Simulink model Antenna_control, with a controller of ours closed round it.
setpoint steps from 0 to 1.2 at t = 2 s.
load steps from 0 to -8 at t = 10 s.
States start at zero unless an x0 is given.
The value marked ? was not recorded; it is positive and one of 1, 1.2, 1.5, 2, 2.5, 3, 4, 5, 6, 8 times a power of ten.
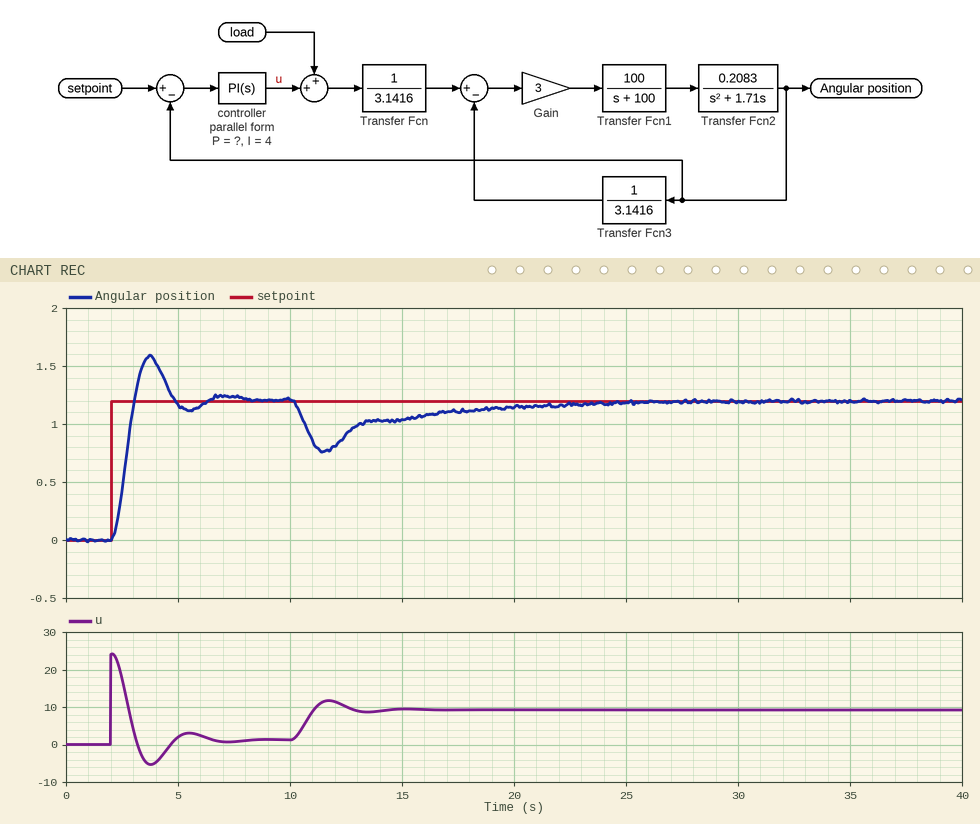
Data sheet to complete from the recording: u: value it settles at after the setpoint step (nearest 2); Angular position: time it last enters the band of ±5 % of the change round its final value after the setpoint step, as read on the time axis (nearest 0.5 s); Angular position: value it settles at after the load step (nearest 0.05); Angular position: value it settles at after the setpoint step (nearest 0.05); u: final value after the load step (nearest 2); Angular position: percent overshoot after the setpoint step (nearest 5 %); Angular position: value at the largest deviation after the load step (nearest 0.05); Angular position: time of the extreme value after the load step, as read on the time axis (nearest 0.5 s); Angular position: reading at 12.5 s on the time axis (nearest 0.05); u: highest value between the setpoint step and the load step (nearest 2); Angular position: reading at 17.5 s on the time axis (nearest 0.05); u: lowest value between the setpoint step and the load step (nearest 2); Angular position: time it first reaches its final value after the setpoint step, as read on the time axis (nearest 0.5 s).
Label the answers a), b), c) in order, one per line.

a) 2
b) 6.0 s
c) 1.20
d) 1.20
e) 10
f) 30 %
g) 0.75
h) 11.5 s
i) 0.90
j) 24
k) 1.10
l) -6
m) 3.0 s
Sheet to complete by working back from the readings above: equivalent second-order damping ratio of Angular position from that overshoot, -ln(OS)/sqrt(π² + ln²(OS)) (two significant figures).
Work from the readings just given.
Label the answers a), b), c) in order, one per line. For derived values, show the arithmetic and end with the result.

a) ln(0.3) = -1.204; 1.204 / sqrt(9.870 + 1.450) = 0.36
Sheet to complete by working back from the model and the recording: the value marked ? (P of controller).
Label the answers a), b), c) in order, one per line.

a) 20
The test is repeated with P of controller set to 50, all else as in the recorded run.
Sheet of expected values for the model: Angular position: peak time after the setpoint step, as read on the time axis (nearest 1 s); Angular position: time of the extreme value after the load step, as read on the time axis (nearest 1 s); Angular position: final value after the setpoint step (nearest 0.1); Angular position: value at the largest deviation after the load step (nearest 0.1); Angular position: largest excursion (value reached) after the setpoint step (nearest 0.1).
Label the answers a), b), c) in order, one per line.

a) 3 s
b) 11 s
c) 1.2
d) 1.0
e) 1.7
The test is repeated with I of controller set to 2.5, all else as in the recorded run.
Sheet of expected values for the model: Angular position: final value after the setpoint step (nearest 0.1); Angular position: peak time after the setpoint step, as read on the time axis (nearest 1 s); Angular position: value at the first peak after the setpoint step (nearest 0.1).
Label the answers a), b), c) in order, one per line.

a) 1.2
b) 4 s
c) 1.5
